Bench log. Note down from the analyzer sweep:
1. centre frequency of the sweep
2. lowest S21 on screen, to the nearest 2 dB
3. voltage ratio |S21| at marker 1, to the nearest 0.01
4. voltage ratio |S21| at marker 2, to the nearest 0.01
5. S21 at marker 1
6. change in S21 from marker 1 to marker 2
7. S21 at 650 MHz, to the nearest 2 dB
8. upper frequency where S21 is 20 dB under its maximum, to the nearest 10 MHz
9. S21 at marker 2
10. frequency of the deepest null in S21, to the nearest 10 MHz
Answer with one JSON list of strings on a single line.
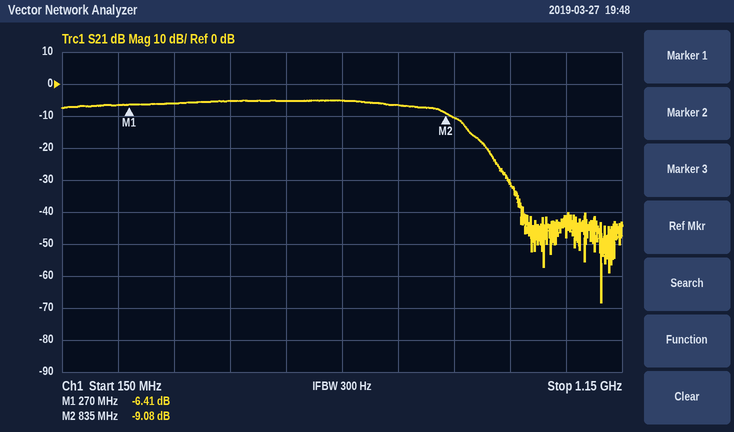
["650 MHz", "-68 dB", "0.48", "0.35", "-6.41 dB", "-2.67 dB", "-6 dB", "930 MHz", "-9.08 dB", "1.11 GHz"]
